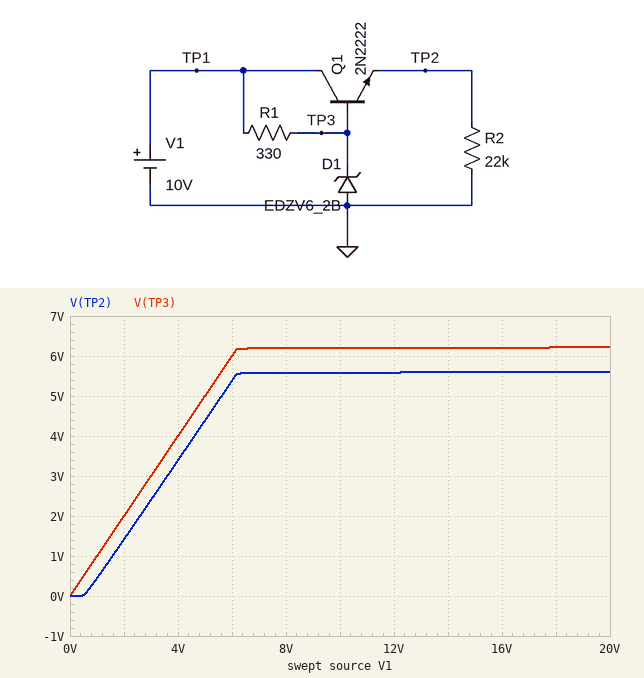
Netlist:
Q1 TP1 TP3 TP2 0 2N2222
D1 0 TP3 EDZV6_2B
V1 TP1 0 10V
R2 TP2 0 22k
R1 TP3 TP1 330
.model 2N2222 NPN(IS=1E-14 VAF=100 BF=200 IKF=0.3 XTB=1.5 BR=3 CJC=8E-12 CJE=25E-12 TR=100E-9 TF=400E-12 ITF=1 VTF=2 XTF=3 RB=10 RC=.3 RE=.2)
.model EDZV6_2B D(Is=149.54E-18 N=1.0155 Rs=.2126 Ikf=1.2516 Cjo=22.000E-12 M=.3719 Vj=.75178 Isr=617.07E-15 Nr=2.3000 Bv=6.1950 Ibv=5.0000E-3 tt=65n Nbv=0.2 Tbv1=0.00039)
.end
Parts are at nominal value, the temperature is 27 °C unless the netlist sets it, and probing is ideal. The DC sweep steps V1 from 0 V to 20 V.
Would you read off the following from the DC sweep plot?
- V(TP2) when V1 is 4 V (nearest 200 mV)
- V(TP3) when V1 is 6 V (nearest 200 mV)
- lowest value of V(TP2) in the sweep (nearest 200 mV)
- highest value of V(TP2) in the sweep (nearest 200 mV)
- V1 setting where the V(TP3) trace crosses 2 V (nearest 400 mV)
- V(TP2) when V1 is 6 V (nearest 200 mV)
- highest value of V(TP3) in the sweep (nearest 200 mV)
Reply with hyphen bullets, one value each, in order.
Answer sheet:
- 3.4 V
- 6.0 V
- 0 V
- 5.6 V
- 2.0 V
- 5.4 V
- 6.2 V
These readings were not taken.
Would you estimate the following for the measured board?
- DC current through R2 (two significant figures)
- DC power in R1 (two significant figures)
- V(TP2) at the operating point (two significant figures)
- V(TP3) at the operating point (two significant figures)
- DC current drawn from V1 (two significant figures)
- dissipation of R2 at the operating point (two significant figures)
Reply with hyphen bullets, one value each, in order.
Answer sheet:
- 250 µA
- 44 mW
- 5.6 V
- 6.2 V
- 12 mA
- 1.4 mW
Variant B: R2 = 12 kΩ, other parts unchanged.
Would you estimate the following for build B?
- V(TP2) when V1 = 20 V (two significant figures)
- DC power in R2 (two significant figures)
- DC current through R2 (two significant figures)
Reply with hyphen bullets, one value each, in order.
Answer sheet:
- 5.6 V
- 2.6 mW
- 460 µA
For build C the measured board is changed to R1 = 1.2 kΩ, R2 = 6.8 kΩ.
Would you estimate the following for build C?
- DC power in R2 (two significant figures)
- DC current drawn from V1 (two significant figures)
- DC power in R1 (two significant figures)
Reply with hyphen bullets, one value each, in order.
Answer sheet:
- 4.5 mW
- 4.0 mA
- 12 mW
